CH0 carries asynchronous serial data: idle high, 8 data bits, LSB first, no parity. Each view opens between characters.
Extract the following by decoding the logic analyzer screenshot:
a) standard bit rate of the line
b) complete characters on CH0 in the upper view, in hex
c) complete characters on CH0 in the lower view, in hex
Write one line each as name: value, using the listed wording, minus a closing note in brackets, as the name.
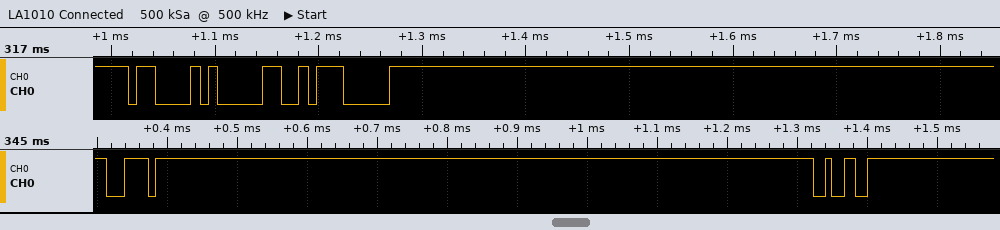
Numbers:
standard bit rate of the line: 115200 baud
complete characters on CH0 in the upper view, in hex: 43, 30, 07
complete characters on CH0 in the lower view, in hex: BC, 32
